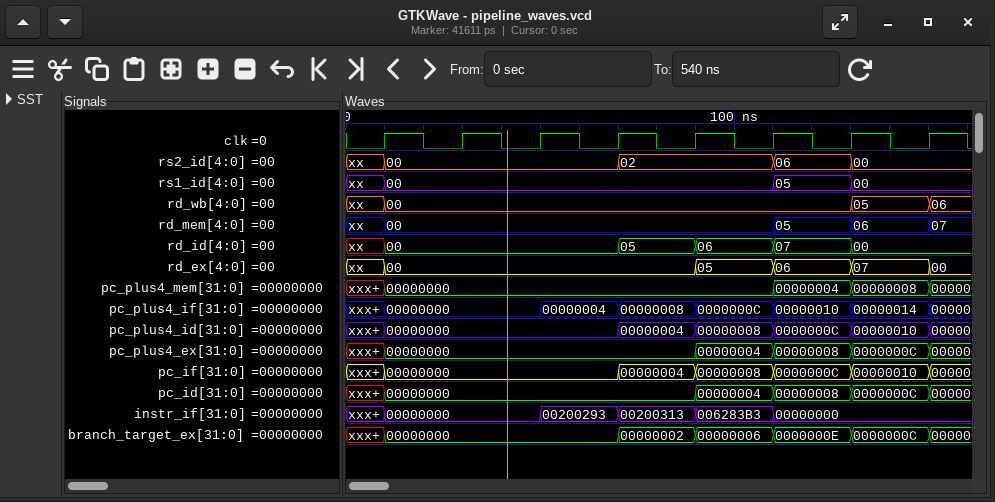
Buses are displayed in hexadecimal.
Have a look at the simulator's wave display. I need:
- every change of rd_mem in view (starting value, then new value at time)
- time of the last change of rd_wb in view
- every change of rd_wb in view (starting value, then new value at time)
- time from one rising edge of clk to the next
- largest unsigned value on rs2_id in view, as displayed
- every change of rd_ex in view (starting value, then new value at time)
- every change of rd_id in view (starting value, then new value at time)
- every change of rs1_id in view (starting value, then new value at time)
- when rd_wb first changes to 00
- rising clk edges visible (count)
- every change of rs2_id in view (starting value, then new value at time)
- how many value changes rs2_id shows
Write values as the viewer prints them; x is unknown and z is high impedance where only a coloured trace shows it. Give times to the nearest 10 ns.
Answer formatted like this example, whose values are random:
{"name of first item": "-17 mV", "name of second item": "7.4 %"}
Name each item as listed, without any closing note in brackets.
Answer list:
{"every change of rd_mem in view": "xx, 00 at 10 ns, 05 at 110 ns, 06 at 130 ns, 07 at 150 ns", "time of the last change of rd_wb in view": "150 ns", "every change of rd_wb in view": "xx, 00 at 10 ns, 05 at 130 ns, 06 at 150 ns", "time from one rising edge of clk to the next": "20 ns", "largest unsigned value on rs2_id in view, as displayed": "06", "every change of rd_ex in view": "xx, 00 at 10 ns, 05 at 90 ns, 06 at 110 ns, 07 at 130 ns, 00 at 150 ns", "every change of rd_id in view": "xx, 00 at 10 ns, 05 at 70 ns, 06 at 90 ns, 07 at 110 ns, 00 at 130 ns", "every change of rs1_id in view": "xx, 00 at 10 ns, 05 at 110 ns, 00 at 130 ns", "when rd_wb first changes to 00": "10 ns", "rising clk edges visible": "8", "every change of rs2_id in view": "xx, 00 at 10 ns, 02 at 70 ns, 06 at 110 ns, 00 at 130 ns", "how many value changes rs2_id shows": "4"}
